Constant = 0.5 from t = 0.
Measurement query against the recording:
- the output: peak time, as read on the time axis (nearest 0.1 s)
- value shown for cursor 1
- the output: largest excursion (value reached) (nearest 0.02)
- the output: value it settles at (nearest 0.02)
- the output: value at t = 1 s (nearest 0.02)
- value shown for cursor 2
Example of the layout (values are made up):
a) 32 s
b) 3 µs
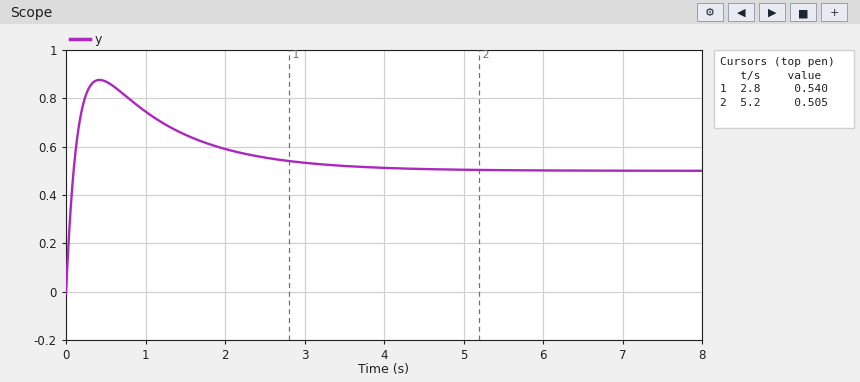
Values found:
a) 0.4 s
b) 0.540
c) 0.88
d) 0.50
e) 0.74
f) 0.505
